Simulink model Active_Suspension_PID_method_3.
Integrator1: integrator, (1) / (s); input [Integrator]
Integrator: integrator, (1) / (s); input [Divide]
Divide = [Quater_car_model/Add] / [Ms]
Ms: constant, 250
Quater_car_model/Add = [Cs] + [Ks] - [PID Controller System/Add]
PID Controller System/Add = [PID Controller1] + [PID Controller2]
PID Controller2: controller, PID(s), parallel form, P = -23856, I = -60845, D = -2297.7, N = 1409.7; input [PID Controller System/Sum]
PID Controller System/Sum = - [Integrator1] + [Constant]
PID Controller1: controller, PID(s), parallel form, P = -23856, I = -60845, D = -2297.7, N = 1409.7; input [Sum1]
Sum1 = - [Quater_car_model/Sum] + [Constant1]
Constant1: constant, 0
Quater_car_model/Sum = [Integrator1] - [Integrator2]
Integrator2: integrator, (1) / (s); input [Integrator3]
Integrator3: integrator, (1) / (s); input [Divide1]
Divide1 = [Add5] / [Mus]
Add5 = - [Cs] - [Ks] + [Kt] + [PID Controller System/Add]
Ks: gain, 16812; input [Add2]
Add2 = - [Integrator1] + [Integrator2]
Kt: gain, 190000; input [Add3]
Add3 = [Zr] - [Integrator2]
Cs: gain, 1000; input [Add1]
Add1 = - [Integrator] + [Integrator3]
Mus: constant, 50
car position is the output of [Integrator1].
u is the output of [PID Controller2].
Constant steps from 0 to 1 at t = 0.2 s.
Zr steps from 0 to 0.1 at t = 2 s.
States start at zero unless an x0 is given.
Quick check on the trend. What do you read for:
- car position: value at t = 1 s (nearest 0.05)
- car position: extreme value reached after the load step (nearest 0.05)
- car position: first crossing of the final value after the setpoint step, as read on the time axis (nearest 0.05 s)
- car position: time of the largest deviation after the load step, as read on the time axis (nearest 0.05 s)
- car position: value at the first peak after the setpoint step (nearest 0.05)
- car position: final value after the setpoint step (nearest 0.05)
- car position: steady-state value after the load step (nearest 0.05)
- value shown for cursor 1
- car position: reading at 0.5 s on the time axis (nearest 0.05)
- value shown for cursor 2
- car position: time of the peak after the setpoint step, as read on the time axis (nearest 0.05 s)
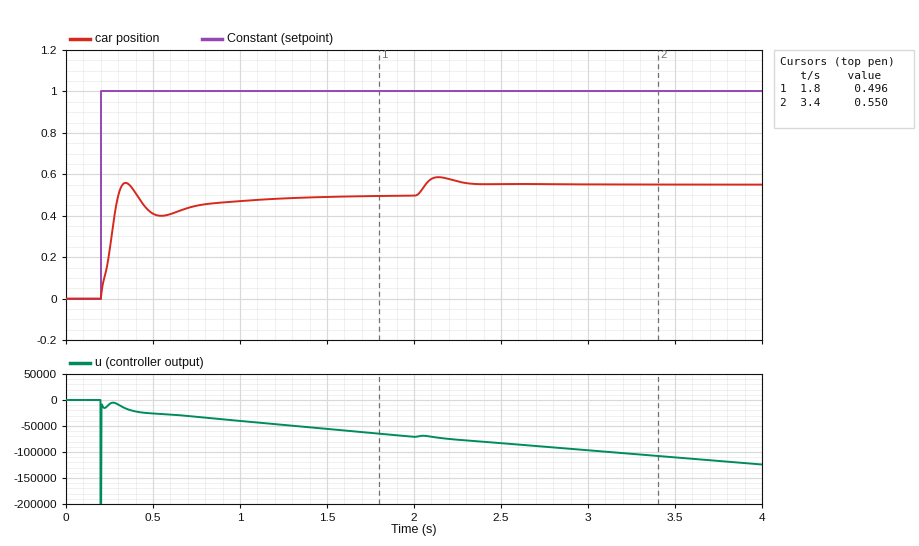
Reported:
0.45
0.60
0.30 s
2.15 s
0.55
0.50
0.55
0.496
0.40
0.550
0.35 s
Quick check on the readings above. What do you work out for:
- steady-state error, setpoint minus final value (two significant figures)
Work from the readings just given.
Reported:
0.50
